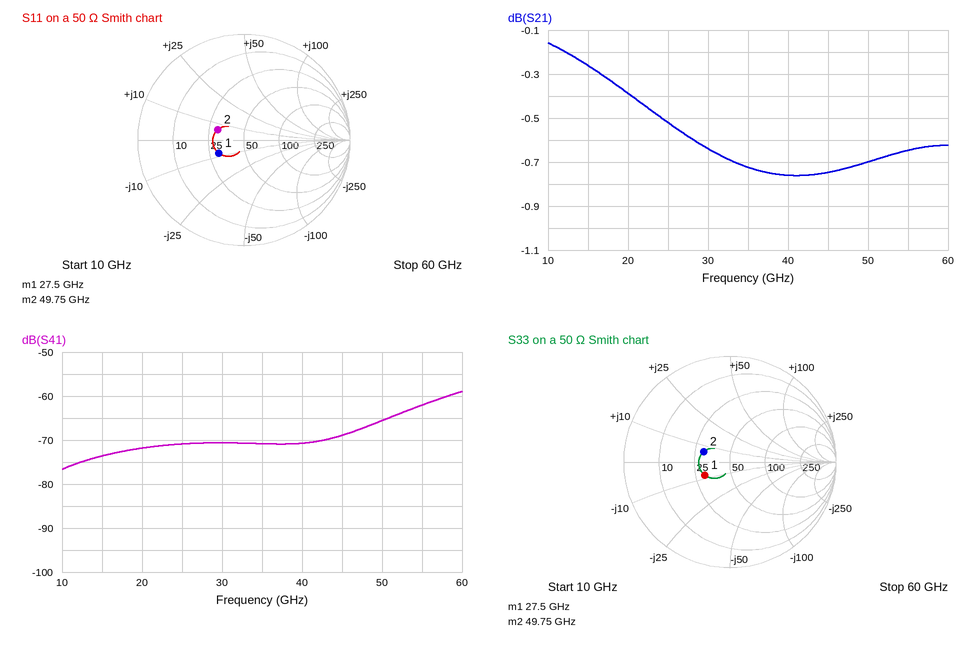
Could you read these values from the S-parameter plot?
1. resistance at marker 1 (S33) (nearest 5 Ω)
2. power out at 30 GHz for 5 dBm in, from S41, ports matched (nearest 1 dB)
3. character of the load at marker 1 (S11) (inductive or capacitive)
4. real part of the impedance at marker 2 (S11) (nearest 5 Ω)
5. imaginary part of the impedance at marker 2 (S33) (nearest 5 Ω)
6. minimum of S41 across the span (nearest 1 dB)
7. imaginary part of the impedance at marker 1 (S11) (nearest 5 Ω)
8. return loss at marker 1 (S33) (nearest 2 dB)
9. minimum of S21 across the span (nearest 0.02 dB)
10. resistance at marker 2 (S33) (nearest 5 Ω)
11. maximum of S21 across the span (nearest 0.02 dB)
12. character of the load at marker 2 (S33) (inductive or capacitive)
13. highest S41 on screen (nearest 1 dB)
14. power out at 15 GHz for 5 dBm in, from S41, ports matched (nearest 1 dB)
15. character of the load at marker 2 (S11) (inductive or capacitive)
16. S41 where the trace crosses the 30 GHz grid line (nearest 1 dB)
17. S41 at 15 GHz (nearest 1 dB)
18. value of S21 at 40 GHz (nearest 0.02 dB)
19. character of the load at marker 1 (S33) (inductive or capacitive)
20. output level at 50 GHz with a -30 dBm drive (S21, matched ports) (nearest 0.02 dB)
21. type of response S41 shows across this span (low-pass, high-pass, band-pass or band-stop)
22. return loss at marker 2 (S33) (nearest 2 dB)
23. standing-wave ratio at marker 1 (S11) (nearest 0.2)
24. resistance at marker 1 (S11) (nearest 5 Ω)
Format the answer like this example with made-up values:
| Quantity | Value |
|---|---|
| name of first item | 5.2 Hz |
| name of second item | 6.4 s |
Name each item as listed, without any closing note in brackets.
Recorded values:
| Quantity | Value |
|---|---|
| resistance at marker 1 (S33) | 30 Ω |
| power out at 30 GHz for 5 dBm in, from S41, ports matched | -66 dBm |
| character of the load at marker 1 (S11) | capacitive |
| real part of the impedance at marker 2 (S11) | 30 Ω |
| imaginary part of the impedance at marker 2 (S33) | +5 Ω |
| minimum of S41 across the span | -77 dB |
| imaginary part of the impedance at marker 1 (S11) | -10 Ω |
| return loss at marker 1 (S33) | 12 dB |
| minimum of S21 across the span | -0.76 dB |
| resistance at marker 2 (S33) | 30 Ω |
| maximum of S21 across the span | -0.16 dB |
| character of the load at marker 2 (S33) | inductive |
| highest S41 on screen | -59 dB |
| power out at 15 GHz for 5 dBm in, from S41, ports matched | -69 dBm |
| character of the load at marker 2 (S11) | inductive |
| S41 where the trace crosses the 30 GHz grid line | -71 dB |
| S41 at 15 GHz | -74 dB |
| value of S21 at 40 GHz | -0.76 dB |
| character of the load at marker 1 (S33) | capacitive |
| output level at 50 GHz with a -30 dBm drive (S21, matched ports) | -30.70 dBm |
| type of response S41 shows across this span | high-pass |
| return loss at marker 2 (S33) | 12 dB |
| standing-wave ratio at marker 1 (S11) | 1.8 |
| resistance at marker 1 (S11) | 30 Ω |
